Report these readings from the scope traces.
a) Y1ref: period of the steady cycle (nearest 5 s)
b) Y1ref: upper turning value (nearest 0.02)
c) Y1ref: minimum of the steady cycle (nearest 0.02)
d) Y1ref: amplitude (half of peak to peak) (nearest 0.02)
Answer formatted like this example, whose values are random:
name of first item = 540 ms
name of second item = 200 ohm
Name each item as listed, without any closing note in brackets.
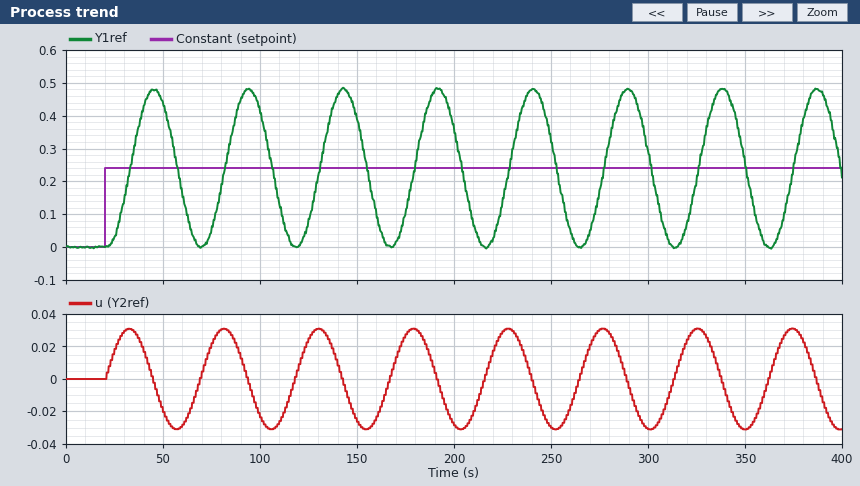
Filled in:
Y1ref: period of the steady cycle = 50 s
Y1ref: upper turning value = 0.48
Y1ref: minimum of the steady cycle = 0.00
Y1ref: amplitude (half of peak to peak) = 0.24
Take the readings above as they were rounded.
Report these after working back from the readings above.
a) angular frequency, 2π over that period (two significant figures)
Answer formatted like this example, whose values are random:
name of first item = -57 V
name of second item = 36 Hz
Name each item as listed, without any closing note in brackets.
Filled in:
angular frequency, 2π over that period = 0.13 rad/s
